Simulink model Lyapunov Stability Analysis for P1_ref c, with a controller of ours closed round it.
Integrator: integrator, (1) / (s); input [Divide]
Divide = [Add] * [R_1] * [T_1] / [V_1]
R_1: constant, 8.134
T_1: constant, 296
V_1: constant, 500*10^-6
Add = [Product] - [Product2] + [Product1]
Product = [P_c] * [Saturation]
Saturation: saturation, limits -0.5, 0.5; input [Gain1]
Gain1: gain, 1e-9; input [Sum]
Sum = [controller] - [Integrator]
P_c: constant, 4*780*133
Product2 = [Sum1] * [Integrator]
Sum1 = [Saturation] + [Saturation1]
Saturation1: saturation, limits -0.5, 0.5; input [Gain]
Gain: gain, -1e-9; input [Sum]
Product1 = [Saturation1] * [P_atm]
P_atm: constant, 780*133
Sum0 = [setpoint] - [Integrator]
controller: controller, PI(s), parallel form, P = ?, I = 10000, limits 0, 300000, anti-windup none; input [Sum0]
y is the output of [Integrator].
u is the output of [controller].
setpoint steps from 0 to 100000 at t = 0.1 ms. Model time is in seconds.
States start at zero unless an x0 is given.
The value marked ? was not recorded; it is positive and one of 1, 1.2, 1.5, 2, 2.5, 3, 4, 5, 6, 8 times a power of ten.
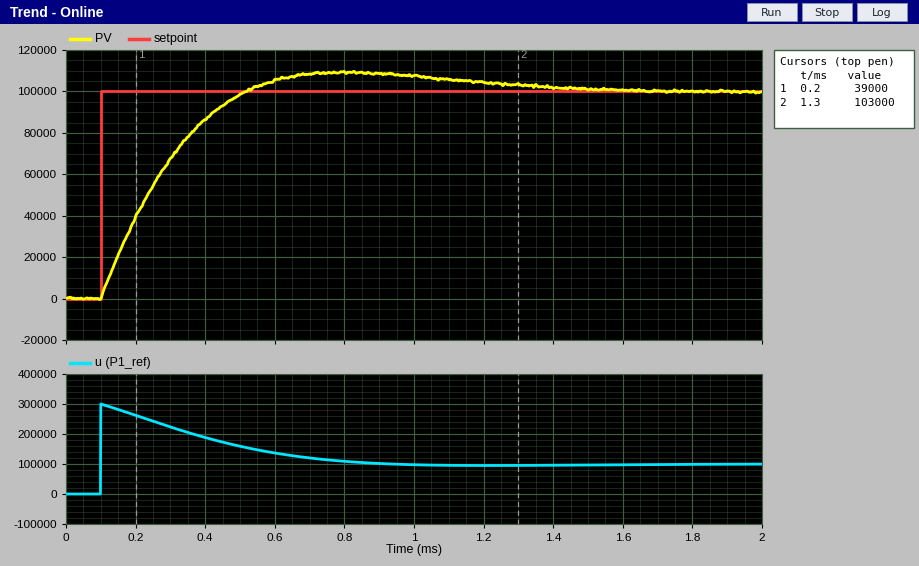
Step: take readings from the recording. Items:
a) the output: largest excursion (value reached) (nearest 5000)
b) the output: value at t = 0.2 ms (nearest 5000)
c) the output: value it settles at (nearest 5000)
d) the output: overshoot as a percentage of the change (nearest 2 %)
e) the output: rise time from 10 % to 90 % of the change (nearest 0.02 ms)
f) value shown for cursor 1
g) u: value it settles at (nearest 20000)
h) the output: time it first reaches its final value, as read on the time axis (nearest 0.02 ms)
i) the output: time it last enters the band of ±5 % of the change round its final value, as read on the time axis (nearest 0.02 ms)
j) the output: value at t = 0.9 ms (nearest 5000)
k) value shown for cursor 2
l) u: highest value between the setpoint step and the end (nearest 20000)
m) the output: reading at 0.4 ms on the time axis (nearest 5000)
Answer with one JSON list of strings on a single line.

["110000", "40000", "100000", "10 %", "0.30 ms", "39000", "100000", "0.52 ms", "1.16 ms", "110000", "103000", "300000", "85000"]
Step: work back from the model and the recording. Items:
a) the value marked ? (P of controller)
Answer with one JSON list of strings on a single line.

["3"]
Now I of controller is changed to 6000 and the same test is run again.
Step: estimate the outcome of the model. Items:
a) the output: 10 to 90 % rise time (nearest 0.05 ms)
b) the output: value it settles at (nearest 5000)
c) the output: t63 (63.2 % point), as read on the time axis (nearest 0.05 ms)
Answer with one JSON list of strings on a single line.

["0.40 ms", "100000", "0.30 ms"]
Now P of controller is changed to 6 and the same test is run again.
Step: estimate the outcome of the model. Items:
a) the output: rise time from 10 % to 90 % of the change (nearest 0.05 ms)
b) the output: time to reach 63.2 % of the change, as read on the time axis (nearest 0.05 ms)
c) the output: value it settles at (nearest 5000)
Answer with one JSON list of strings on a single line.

["0.25 ms", "0.25 ms", "100000"]
